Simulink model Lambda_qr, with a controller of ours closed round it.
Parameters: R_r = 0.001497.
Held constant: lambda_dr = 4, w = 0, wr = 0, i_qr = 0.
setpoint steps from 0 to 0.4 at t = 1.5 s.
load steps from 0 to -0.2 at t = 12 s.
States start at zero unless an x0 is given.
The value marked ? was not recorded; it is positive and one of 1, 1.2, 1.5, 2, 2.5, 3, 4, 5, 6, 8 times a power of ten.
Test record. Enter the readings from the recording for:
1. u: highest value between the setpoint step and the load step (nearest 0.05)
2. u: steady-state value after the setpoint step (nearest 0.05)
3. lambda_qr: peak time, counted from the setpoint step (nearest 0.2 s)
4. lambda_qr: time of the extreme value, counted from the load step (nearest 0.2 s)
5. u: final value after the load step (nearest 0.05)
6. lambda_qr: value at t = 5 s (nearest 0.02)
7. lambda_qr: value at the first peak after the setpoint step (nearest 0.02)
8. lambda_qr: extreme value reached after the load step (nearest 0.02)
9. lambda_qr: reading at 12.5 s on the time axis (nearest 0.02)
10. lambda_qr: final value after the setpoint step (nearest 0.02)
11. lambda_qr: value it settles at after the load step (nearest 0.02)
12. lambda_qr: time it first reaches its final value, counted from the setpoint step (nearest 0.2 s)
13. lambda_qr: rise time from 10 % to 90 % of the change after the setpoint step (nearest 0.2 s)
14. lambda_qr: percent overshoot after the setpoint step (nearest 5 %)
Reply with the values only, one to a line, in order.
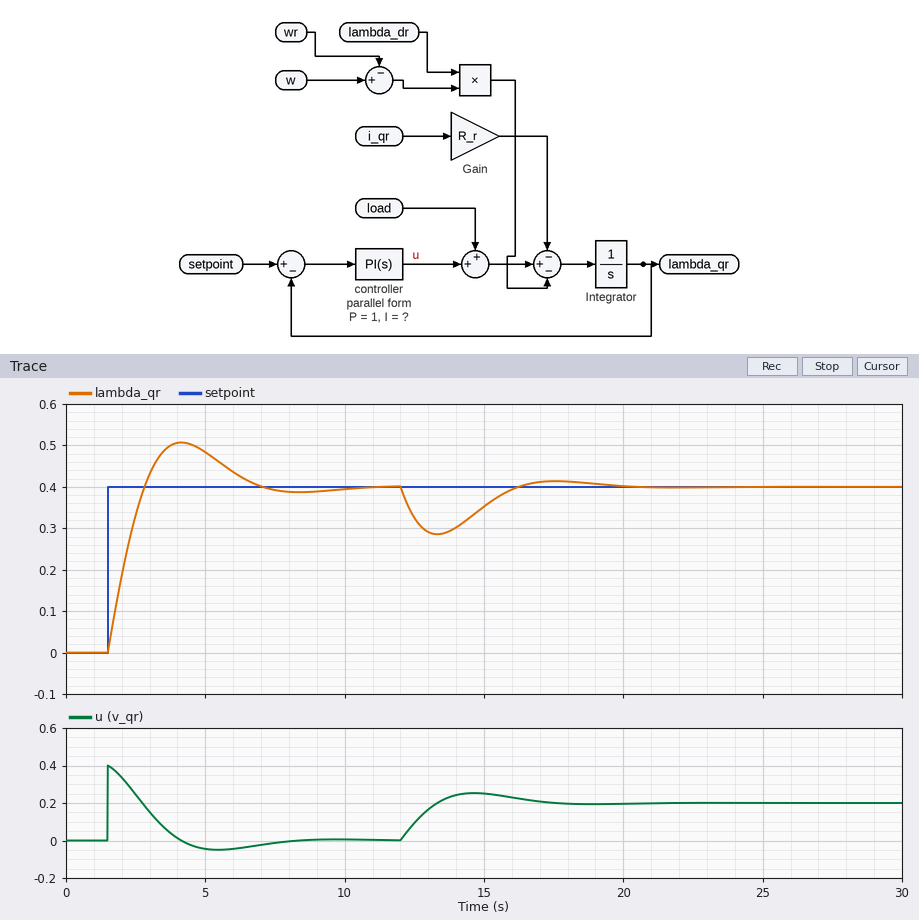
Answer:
0.40
0.00
2.6 s
1.4 s
0.20
0.48
0.50
0.28
0.32
0.40
0.40
1.4 s
1.0 s
25 %
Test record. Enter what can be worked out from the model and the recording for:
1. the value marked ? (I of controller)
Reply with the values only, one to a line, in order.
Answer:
0.8
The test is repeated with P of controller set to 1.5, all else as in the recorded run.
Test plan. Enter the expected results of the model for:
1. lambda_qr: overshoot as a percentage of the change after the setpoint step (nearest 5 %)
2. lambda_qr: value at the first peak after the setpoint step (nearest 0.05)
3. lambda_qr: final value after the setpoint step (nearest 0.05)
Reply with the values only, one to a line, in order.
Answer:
15 %
0.45
0.40
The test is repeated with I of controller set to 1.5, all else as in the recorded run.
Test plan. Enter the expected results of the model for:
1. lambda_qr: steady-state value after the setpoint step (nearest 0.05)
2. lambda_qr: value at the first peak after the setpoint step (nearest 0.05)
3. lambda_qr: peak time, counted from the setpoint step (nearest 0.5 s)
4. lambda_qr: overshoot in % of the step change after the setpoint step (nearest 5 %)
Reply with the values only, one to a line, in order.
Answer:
0.40
0.55
2.0 s
35 %
